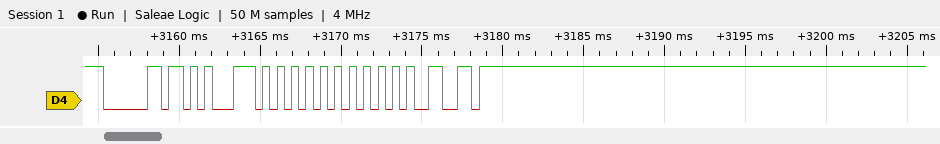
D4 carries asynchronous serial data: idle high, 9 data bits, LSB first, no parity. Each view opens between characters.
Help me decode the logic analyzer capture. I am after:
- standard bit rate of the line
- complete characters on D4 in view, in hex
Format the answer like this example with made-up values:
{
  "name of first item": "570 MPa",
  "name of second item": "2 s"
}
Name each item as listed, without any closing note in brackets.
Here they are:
{
  "standard bit rate of the line": "2400 baud",
  "complete characters on D4 in view, in hex": "E0, 1C5, D5, D5, 119, 1FF"
}
